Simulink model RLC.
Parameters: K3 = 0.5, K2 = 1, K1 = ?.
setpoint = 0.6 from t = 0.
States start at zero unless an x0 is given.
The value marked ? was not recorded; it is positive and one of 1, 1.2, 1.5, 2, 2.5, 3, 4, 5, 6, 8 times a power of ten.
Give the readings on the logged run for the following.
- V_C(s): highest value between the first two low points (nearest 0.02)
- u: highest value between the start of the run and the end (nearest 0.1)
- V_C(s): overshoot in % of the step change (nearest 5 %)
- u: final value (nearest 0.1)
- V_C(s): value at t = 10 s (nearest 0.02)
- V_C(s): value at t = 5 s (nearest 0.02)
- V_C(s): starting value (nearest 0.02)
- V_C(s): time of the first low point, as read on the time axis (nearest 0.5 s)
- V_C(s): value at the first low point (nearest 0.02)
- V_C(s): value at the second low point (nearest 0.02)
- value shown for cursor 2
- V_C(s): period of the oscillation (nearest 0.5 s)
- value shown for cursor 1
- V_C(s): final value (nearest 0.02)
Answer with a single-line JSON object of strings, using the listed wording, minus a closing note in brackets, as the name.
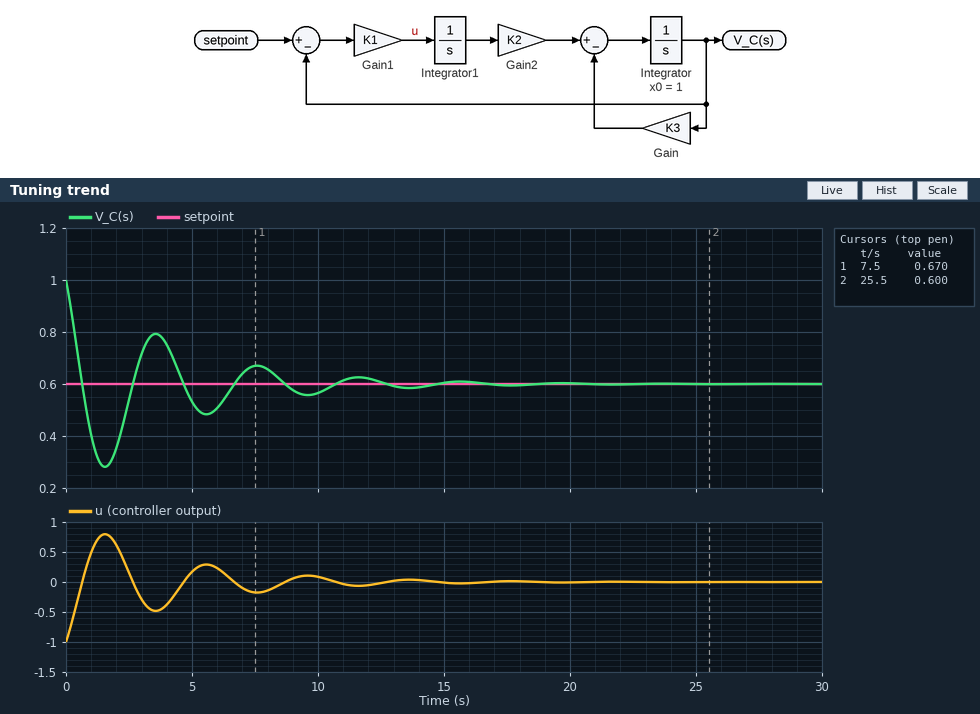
{"V_C(s): highest value between the first two low points": "0.80", "u: highest value between the start of the run and the end": "0.8", "V_C(s): overshoot in % of the step change": "80 %", "u: final value": "0.0", "V_C(s): value at t = 10 s": "0.56", "V_C(s): value at t = 5 s": "0.54", "V_C(s): starting value": "1.00", "V_C(s): time of the first low point, as read on the time axis": "1.5 s", "V_C(s): value at the first low point": "0.28", "V_C(s): value at the second low point": "0.48", "value shown for cursor 2": "0.600", "V_C(s): period of the oscillation": "4.0 s", "value shown for cursor 1": "0.670", "V_C(s): final value": "0.60"}
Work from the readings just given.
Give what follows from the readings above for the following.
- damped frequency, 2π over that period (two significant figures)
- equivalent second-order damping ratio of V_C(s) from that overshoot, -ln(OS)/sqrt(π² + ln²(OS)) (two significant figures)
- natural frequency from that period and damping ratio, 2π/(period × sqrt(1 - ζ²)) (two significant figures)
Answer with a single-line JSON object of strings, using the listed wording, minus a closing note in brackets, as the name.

{"damped frequency, 2π over that period": "1.6 rad/s", "equivalent second-order damping ratio of V_C(s) from that overshoot, -ln(OS)/sqrt(π² + ln²(OS))": "0.071", "natural frequency from that period and damping ratio, 2π/(period × sqrt(1 - ζ²))": "1.6 rad/s"}
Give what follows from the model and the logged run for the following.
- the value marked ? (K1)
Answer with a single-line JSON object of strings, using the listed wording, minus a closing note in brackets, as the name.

{"the value marked ?": "2.5"}
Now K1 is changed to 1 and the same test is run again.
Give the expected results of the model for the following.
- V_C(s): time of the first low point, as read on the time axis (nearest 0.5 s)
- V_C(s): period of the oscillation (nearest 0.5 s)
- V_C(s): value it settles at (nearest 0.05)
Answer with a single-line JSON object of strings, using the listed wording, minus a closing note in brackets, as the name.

{"V_C(s): time of the first low point, as read on the time axis": "2.0 s", "V_C(s): period of the oscillation": "6.5 s", "V_C(s): value it settles at": "0.60"}
